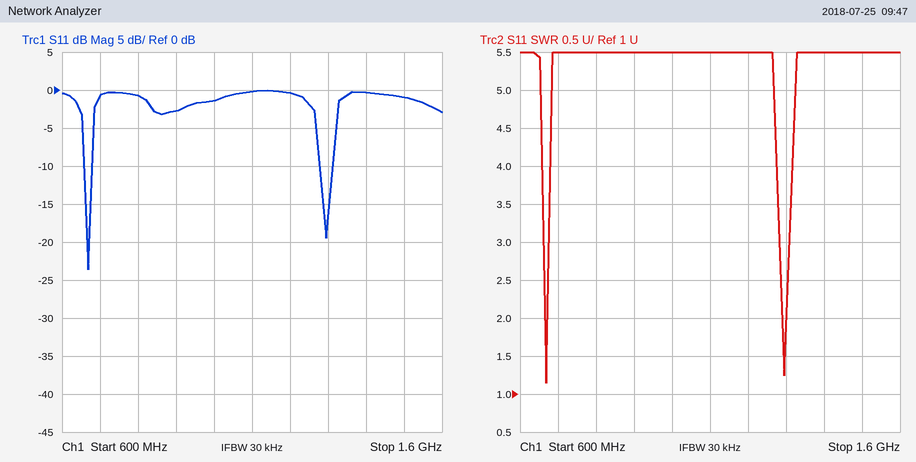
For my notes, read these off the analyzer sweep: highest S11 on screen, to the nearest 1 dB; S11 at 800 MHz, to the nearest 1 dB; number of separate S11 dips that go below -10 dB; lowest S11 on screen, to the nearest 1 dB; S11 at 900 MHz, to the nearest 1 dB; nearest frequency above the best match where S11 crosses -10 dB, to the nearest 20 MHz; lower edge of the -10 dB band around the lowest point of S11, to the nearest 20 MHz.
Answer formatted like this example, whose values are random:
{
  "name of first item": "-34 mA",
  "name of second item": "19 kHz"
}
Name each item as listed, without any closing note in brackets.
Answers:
{
  "highest S11 on screen, to the nearest 1 dB": "0 dB",
  "S11 at 800 MHz, to the nearest 1 dB": "-1 dB",
  "number of separate S11 dips that go below -10 dB": "2",
  "lowest S11 on screen, to the nearest 1 dB": "-24 dB",
  "S11 at 900 MHz, to the nearest 1 dB": "-3 dB",
  "nearest frequency above the best match where S11 crosses -10 dB, to the nearest 20 MHz": "680 MHz",
  "lower edge of the -10 dB band around the lowest point of S11, to the nearest 20 MHz": "660 MHz"
}
